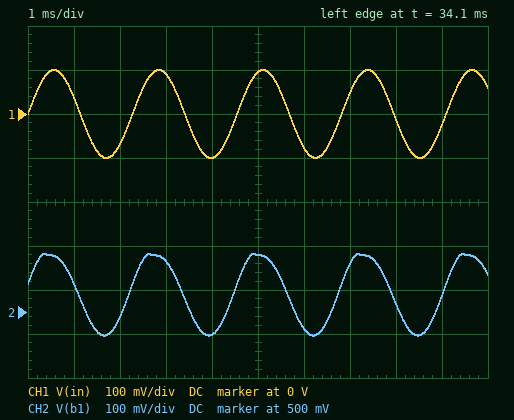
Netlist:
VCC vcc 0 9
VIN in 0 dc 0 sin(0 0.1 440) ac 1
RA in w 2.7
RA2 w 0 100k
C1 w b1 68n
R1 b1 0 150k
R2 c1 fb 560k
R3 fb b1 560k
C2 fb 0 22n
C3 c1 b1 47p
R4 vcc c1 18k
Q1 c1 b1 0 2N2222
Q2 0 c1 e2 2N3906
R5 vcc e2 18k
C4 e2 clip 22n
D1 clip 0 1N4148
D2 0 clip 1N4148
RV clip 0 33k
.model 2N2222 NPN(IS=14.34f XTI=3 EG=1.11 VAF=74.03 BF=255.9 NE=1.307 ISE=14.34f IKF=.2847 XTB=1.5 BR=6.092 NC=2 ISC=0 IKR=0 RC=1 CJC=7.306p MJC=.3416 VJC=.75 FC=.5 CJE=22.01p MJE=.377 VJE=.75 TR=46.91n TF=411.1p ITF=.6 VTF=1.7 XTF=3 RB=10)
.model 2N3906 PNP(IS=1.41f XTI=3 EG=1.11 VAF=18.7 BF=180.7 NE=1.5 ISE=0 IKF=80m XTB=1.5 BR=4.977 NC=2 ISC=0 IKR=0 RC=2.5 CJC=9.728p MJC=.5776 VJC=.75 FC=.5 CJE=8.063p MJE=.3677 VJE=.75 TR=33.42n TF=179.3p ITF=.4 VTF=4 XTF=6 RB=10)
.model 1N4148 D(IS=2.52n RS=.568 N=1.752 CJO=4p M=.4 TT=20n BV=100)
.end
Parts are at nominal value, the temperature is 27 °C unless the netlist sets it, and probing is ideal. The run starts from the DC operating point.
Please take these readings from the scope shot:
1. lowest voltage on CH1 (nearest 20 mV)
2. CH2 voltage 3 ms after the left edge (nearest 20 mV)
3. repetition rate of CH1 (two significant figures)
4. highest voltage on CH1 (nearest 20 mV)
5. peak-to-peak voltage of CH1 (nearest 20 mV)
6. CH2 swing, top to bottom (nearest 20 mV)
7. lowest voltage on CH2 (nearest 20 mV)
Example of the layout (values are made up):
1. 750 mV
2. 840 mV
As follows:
1. -100 mV
2. 620 mV
3. 440 Hz
4. 100 mV
5. 200 mV
6. 180 mV
7. 440 mV
